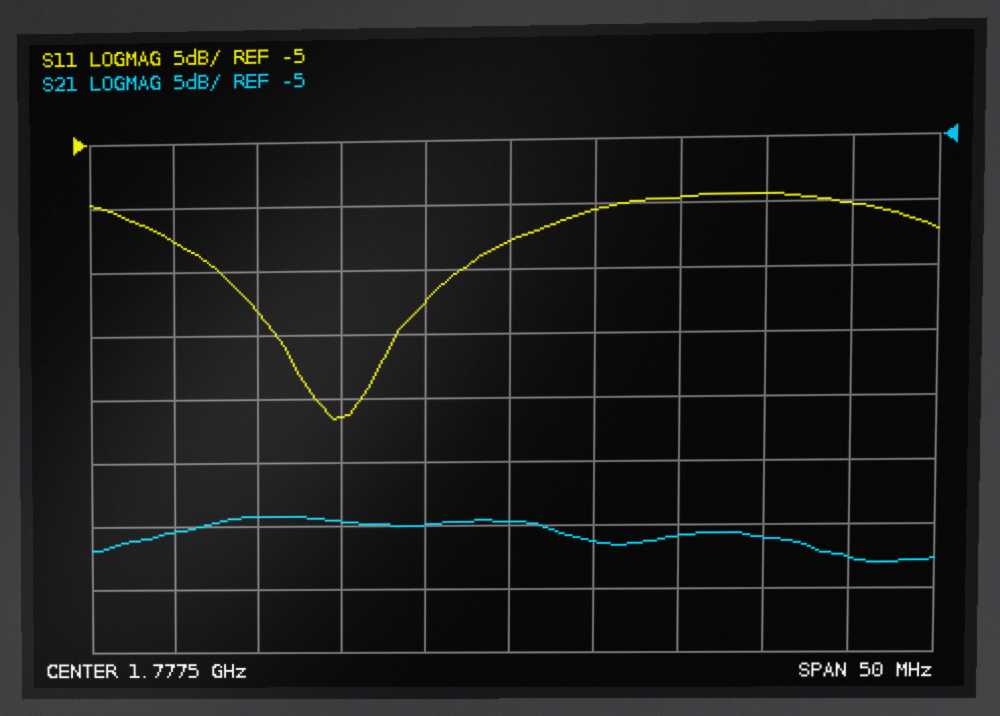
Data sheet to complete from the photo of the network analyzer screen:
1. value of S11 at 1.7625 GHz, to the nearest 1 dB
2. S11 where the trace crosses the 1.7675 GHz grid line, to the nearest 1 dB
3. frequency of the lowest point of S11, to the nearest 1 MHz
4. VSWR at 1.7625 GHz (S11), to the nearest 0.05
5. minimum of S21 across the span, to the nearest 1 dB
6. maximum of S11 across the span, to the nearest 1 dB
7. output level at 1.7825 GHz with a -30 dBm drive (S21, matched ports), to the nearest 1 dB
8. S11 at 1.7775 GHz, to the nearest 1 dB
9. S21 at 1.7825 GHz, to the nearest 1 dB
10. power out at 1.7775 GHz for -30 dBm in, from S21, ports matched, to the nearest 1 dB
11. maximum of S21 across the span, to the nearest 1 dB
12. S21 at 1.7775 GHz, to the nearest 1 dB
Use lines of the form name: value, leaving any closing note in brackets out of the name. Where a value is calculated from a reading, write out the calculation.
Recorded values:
value of S11 at 1.7625 GHz, to the nearest 1 dB: -18 dB
S11 where the trace crosses the 1.7675 GHz grid line, to the nearest 1 dB: -26 dB
frequency of the lowest point of S11, to the nearest 1 MHz: 1.767 GHz
VSWR at 1.7625 GHz (S11), to the nearest 0.05: |Γ| = 10^(-18/20) = 0.1259; VSWR = (1 + 0.1259)/(1 − 0.1259) ≈ 1.29, so 1.30 to the nearest 0.05
minimum of S21 across the span, to the nearest 1 dB: -38 dB
maximum of S11 across the span, to the nearest 1 dB: -9 dB
output level at 1.7825 GHz with a -30 dBm drive (S21, matched ports), to the nearest 1 dB: -30 dBm + (-36 dB) = -66 dBm
S11 at 1.7775 GHz, to the nearest 1 dB: -13 dB
S21 at 1.7825 GHz, to the nearest 1 dB: -36 dB
power out at 1.7775 GHz for -30 dBm in, from S21, ports matched, to the nearest 1 dB: -30 dBm + (-35 dB) = -65 dBm
maximum of S21 across the span, to the nearest 1 dB: -34 dB
S21 at 1.7775 GHz, to the nearest 1 dB: -35 dB
